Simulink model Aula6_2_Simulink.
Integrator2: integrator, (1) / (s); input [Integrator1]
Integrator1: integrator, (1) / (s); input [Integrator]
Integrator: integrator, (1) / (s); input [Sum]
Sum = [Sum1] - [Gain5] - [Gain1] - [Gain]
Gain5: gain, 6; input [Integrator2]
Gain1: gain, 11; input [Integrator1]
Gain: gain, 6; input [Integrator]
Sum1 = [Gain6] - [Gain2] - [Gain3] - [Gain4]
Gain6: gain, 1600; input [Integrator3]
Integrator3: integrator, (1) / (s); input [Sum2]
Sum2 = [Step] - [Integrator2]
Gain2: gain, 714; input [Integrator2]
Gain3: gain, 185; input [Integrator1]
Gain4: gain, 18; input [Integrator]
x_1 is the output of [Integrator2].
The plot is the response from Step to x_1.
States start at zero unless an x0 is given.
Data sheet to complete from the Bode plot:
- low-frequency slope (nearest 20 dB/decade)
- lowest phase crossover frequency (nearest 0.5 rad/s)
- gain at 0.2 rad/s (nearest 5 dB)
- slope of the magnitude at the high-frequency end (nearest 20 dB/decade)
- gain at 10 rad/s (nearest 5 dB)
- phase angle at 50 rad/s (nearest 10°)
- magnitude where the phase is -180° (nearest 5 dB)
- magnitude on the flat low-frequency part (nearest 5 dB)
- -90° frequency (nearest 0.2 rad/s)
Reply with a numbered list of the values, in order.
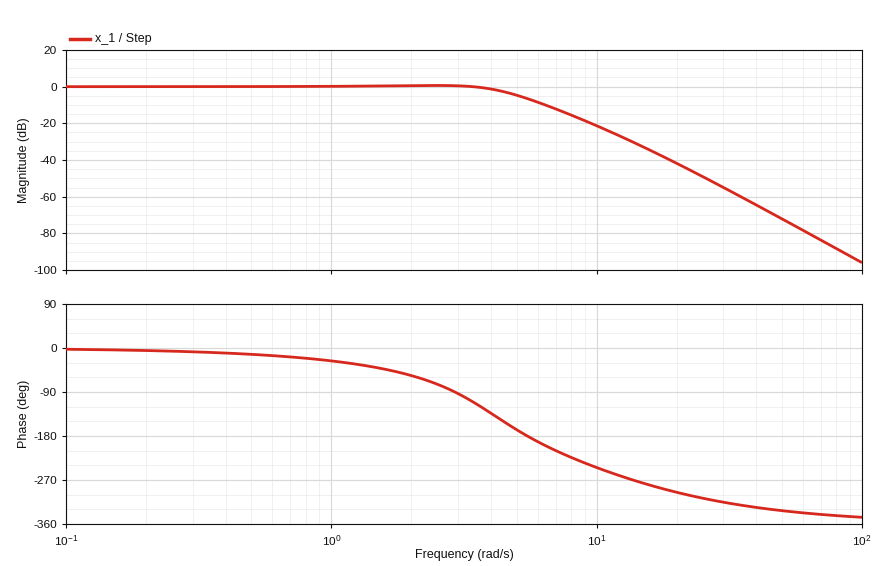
1. 0 dB/decade
2. 5.5 rad/s
3. 0 dB
4. -80 dB/decade
5. -20 dB
6. -330°
7. -5 dB
8. 0 dB
9. 3.0 rad/s
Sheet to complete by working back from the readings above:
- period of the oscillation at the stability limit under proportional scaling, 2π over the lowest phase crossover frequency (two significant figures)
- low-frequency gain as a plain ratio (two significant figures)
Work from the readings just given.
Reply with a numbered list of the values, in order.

1. 1.1 s
2. 1.0
